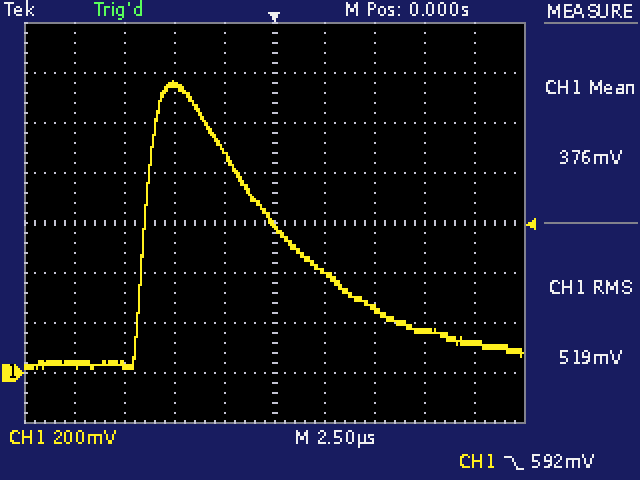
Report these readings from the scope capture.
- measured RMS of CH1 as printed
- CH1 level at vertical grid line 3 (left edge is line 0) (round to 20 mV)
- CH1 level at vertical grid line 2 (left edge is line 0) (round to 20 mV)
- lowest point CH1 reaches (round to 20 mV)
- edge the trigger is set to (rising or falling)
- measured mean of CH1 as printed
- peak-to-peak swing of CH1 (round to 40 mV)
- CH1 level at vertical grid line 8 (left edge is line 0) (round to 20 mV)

519 mV
1.16 V
40 mV
20 mV
falling
376 mV
1.16 V
160 mV
